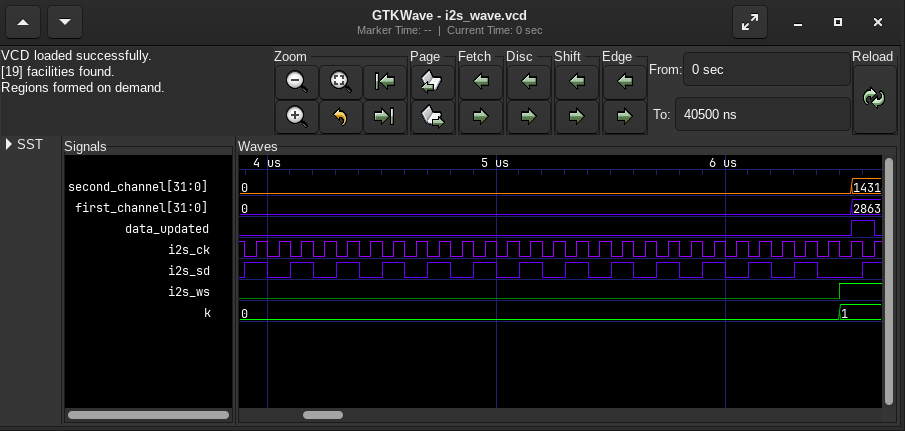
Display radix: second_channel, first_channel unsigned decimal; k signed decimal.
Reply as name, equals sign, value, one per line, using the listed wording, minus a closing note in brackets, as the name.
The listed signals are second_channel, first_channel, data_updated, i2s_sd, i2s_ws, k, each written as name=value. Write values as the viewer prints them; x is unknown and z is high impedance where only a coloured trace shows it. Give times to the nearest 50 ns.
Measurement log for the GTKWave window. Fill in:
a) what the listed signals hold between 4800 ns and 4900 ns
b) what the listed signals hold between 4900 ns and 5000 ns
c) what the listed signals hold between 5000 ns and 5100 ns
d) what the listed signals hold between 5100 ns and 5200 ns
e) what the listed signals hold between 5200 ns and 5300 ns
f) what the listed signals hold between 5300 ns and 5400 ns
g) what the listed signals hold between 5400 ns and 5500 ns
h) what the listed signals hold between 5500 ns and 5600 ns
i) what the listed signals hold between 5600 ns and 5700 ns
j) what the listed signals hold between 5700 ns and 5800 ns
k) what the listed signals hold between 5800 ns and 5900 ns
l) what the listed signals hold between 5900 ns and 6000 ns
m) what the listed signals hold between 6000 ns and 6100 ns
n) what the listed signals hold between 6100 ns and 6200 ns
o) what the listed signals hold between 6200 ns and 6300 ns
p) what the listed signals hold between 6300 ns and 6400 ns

what the listed signals hold between 4800 ns and 4900 ns = second_channel=0, first_channel=0, data_updated=0, i2s_sd=0, i2s_ws=0, k=0
what the listed signals hold between 4900 ns and 5000 ns = second_channel=0, first_channel=0, data_updated=0, i2s_sd=1, i2s_ws=0, k=0
what the listed signals hold between 5000 ns and 5100 ns = second_channel=0, first_channel=0, data_updated=0, i2s_sd=0, i2s_ws=0, k=0
what the listed signals hold between 5100 ns and 5200 ns = second_channel=0, first_channel=0, data_updated=0, i2s_sd=1, i2s_ws=0, k=0
what the listed signals hold between 5200 ns and 5300 ns = second_channel=0, first_channel=0, data_updated=0, i2s_sd=0, i2s_ws=0, k=0
what the listed signals hold between 5300 ns and 5400 ns = second_channel=0, first_channel=0, data_updated=0, i2s_sd=1, i2s_ws=0, k=0
what the listed signals hold between 5400 ns and 5500 ns = second_channel=0, first_channel=0, data_updated=0, i2s_sd=0, i2s_ws=0, k=0
what the listed signals hold between 5500 ns and 5600 ns = second_channel=0, first_channel=0, data_updated=0, i2s_sd=1, i2s_ws=0, k=0
what the listed signals hold between 5600 ns and 5700 ns = second_channel=0, first_channel=0, data_updated=0, i2s_sd=0, i2s_ws=0, k=0
what the listed signals hold between 5700 ns and 5800 ns = second_channel=0, first_channel=0, data_updated=0, i2s_sd=1, i2s_ws=0, k=0
what the listed signals hold between 5800 ns and 5900 ns = second_channel=0, first_channel=0, data_updated=0, i2s_sd=0, i2s_ws=0, k=0
what the listed signals hold between 5900 ns and 6000 ns = second_channel=0, first_channel=0, data_updated=0, i2s_sd=1, i2s_ws=0, k=0
what the listed signals hold between 6000 ns and 6100 ns = second_channel=0, first_channel=0, data_updated=0, i2s_sd=0, i2s_ws=0, k=0
what the listed signals hold between 6100 ns and 6200 ns = second_channel=0, first_channel=0, data_updated=0, i2s_sd=1, i2s_ws=0, k=0
what the listed signals hold between 6200 ns and 6300 ns = second_channel=0, first_channel=0, data_updated=0, i2s_sd=0, i2s_ws=0, k=0
what the listed signals hold between 6300 ns and 6400 ns = second_channel=0, first_channel=0, data_updated=0, i2s_sd=1, i2s_ws=0, k=0
